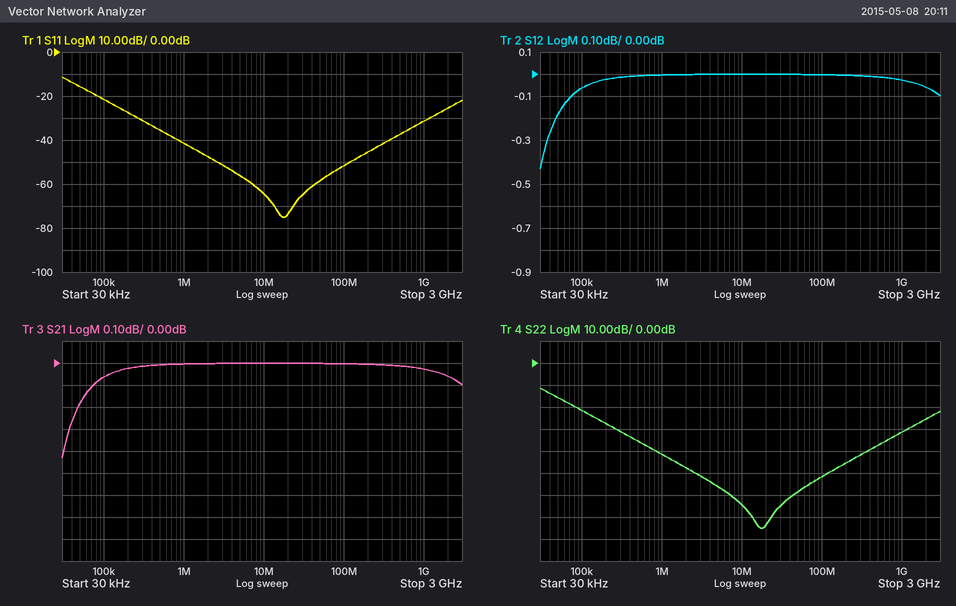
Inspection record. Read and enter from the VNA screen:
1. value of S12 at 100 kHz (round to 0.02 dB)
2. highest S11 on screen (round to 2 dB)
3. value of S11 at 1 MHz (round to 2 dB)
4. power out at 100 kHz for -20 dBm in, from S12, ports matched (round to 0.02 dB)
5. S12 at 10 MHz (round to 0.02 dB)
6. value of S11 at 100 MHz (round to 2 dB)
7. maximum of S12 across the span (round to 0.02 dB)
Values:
-0.06 dB
-12 dB
-42 dB
-20.06 dBm
0.00 dB
-52 dB
0.00 dB
